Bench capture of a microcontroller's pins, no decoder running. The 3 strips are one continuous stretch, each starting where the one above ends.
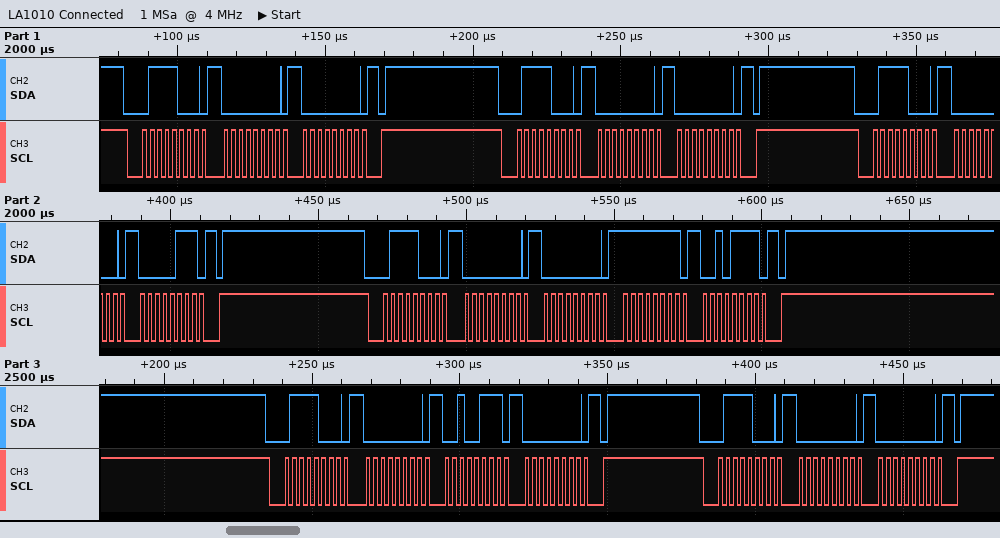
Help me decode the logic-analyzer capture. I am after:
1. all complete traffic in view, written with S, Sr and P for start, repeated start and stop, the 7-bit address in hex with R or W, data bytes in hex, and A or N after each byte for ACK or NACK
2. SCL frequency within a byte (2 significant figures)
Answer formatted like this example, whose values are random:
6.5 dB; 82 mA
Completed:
S 3CW A 00 A 00 A P S 3CW A 00 A 00 A P S 3CW A 00 A 07 A P S 3CW A 00 A 00 A FF A 2F A P S 3CW A 00 A 27 A 00 A P S 3CW A 00 A 00 A P; 400 kHz
